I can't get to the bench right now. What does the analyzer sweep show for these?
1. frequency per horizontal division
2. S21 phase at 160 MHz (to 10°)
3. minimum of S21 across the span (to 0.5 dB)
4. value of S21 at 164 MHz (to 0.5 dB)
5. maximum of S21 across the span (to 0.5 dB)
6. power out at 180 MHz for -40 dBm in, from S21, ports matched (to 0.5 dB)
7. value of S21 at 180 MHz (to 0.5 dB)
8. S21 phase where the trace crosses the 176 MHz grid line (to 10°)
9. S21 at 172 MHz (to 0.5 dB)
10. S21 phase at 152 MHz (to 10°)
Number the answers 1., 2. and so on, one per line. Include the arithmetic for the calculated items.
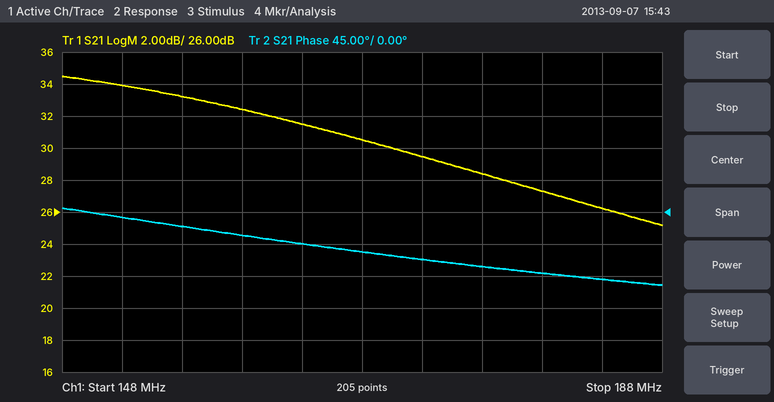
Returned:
1. 4 MHz
2. -30°
3. 25.0 dB
4. 31.5 dB
5. 34.5 dB
6. -40 dBm + (27.5 dB) = -12.5 dBm
7. 27.5 dB
8. -80°
9. 29.5 dB
10. -10°
